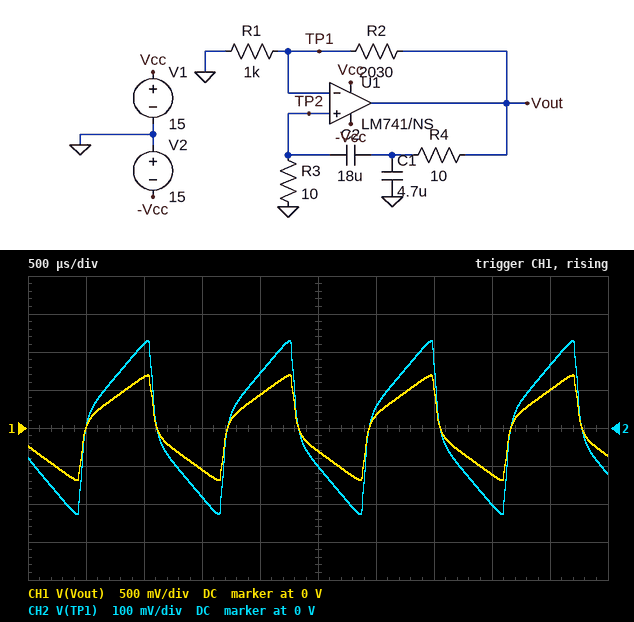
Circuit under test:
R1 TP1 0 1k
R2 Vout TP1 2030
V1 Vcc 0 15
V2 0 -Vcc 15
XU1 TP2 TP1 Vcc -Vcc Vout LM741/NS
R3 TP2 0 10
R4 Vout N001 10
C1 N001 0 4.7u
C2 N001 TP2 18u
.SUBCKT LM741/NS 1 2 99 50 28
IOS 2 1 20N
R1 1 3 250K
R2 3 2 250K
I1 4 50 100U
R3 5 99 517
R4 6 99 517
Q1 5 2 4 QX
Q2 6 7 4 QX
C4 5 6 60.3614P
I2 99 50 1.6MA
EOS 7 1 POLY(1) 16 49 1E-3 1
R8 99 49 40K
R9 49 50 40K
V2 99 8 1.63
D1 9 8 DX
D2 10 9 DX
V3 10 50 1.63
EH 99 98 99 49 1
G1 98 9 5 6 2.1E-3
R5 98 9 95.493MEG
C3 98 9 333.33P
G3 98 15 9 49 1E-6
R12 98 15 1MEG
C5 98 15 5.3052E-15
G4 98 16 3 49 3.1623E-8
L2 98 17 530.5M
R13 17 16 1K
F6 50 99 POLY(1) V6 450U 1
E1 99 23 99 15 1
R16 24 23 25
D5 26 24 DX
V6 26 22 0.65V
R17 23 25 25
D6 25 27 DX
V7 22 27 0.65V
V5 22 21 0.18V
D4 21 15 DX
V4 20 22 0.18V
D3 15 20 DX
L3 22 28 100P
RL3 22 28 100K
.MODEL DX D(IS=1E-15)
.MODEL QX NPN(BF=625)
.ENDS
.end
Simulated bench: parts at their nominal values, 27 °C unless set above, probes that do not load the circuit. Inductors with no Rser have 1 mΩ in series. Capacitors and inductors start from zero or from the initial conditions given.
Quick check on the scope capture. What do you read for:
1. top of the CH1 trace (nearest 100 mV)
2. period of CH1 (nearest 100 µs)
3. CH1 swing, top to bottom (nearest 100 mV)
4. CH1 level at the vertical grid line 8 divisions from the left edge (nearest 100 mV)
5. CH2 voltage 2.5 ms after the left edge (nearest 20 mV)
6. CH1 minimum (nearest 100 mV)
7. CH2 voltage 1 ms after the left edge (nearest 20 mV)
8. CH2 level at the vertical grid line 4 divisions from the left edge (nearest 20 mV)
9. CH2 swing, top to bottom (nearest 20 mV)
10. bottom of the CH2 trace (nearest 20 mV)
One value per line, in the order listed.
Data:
700 mV
1.2 ms
1.4 V
-600 mV
-100 mV
-700 mV
220 mV
140 mV
460 mV
-220 mV
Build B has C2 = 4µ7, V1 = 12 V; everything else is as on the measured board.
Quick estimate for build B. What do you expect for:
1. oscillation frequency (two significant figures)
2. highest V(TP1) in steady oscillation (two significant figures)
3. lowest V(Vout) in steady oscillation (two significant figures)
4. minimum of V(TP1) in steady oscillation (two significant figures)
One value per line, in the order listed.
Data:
2.3 kHz
170 mV
-540 mV
-180 mV
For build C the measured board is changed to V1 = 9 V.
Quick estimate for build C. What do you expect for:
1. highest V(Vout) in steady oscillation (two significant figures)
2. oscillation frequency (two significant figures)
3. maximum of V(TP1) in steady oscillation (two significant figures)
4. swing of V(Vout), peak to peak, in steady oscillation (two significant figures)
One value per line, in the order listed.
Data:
650 mV
850 Hz
210 mV
1.3 V
